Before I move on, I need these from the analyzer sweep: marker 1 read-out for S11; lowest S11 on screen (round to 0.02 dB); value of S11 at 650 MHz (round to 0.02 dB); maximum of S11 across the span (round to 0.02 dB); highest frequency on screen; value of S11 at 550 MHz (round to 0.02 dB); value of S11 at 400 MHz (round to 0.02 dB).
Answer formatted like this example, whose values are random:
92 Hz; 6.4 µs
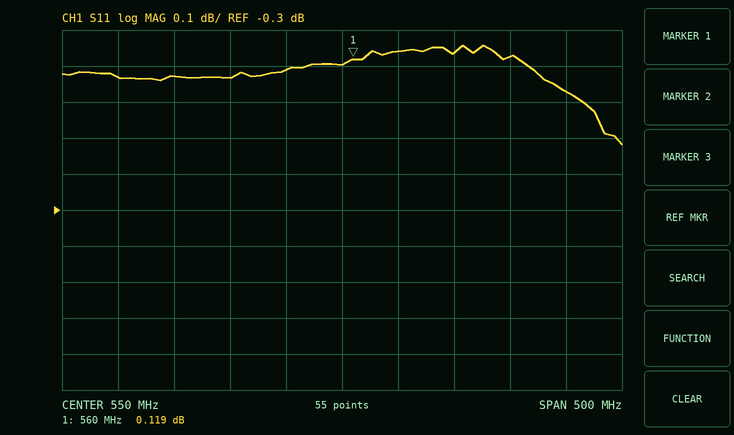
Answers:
0.119 dB; -0.12 dB; 0.14 dB; 0.16 dB; 800 MHz; 0.10 dB; 0.08 dB
